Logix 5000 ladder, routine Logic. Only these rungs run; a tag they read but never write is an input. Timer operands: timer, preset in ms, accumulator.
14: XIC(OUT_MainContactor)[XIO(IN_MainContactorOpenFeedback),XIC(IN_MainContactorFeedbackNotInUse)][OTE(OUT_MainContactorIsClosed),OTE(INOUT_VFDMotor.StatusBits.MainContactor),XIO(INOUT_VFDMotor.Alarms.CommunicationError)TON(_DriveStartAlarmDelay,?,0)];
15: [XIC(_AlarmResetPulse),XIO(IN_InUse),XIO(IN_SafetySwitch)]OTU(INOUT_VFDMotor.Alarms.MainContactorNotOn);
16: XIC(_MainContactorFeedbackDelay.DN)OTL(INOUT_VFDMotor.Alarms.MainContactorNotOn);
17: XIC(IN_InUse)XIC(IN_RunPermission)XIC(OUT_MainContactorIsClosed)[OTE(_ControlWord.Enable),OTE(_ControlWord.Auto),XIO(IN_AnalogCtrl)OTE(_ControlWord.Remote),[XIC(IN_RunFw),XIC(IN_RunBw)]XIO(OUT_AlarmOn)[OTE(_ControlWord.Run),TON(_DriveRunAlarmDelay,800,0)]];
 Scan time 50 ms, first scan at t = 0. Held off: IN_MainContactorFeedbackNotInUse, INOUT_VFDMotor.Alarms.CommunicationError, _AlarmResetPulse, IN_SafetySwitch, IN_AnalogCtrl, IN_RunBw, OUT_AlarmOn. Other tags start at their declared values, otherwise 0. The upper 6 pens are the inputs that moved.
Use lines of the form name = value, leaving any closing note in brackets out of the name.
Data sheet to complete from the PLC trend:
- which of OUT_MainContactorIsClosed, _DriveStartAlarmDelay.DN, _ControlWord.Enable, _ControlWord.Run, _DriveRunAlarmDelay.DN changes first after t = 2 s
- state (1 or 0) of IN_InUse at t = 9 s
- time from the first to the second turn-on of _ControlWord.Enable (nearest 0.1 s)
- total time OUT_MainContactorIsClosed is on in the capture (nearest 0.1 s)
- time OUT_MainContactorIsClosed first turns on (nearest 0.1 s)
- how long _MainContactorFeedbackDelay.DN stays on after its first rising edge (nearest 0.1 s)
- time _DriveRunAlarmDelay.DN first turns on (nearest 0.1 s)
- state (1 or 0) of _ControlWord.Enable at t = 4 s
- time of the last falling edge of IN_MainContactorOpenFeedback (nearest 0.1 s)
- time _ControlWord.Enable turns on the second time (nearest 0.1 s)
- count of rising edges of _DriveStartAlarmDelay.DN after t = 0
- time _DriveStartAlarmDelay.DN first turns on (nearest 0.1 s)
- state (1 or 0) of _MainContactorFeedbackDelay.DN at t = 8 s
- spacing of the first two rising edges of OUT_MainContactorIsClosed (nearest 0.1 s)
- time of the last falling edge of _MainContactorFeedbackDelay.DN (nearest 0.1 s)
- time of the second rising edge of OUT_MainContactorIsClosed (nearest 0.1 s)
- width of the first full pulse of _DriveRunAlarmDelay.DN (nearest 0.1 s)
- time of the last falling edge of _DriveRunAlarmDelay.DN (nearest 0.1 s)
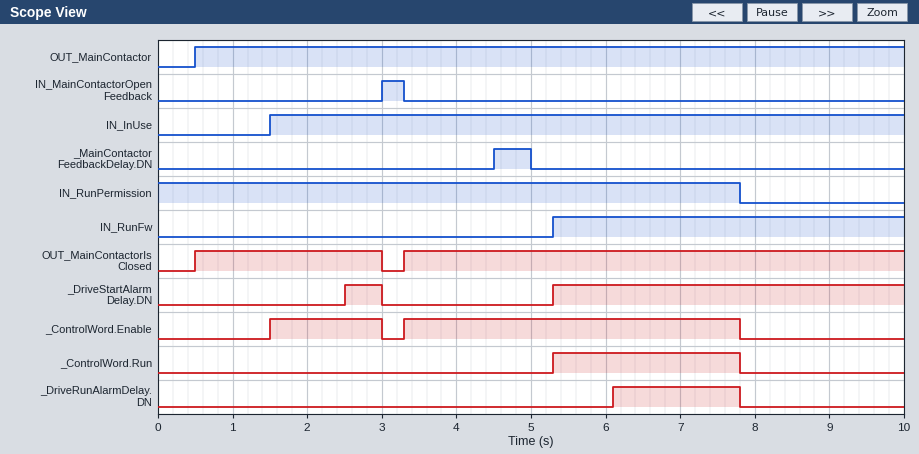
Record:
which of OUT_MainContactorIsClosed, _DriveStartAlarmDelay.DN, _ControlWord.Enable, _ControlWord.Run, _DriveRunAlarmDelay.DN changes first after t = 2 s = _DriveStartAlarmDelay.DN
state (1 or 0) of IN_InUse at t = 9 s = 1
time from the first to the second turn-on of _ControlWord.Enable = 1.8 s
total time OUT_MainContactorIsClosed is on in the capture = 9.2 s
time OUT_MainContactorIsClosed first turns on = 0.5 s
how long _MainContactorFeedbackDelay.DN stays on after its first rising edge = 0.5 s
time _DriveRunAlarmDelay.DN first turns on = 6.1 s
state (1 or 0) of _ControlWord.Enable at t = 4 s = 1
time of the last falling edge of IN_MainContactorOpenFeedback = 3.3 s
time _ControlWord.Enable turns on the second time = 3.3 s
count of rising edges of _DriveStartAlarmDelay.DN after t = 0 = 2
time _DriveStartAlarmDelay.DN first turns on = 2.5 s
state (1 or 0) of _MainContactorFeedbackDelay.DN at t = 8 s = 0
spacing of the first two rising edges of OUT_MainContactorIsClosed = 2.8 s
time of the last falling edge of _MainContactorFeedbackDelay.DN = 5.0 s
time of the second rising edge of OUT_MainContactorIsClosed = 3.3 s
width of the first full pulse of _DriveRunAlarmDelay.DN = 1.7 s
time of the last falling edge of _DriveRunAlarmDelay.DN = 7.8 s
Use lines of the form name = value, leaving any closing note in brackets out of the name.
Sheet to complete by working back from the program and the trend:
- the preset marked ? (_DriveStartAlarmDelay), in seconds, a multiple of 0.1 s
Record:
the preset marked ? (_DriveStartAlarmDelay), in seconds, a multiple of 0.1 s = 2.0 s
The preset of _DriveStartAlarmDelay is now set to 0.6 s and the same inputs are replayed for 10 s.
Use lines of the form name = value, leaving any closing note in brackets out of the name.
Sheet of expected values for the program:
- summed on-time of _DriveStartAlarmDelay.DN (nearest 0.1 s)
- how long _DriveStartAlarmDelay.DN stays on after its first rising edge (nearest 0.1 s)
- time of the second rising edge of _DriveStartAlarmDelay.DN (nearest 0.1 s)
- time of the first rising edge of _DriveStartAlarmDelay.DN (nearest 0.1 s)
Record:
summed on-time of _DriveStartAlarmDelay.DN = 8.0 s
how long _DriveStartAlarmDelay.DN stays on after its first rising edge = 1.9 s
time of the second rising edge of _DriveStartAlarmDelay.DN = 3.9 s
time of the first rising edge of _DriveStartAlarmDelay.DN = 1.1 s
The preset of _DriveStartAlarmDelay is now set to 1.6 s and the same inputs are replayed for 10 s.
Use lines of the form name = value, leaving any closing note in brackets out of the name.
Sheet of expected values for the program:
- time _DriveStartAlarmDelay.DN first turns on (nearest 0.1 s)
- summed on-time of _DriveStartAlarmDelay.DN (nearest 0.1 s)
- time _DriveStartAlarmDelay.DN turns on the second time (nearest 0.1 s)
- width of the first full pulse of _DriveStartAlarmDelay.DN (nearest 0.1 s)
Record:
time _DriveStartAlarmDelay.DN first turns on = 2.1 s
summed on-time of _DriveStartAlarmDelay.DN = 6.0 s
time _DriveStartAlarmDelay.DN turns on the second time = 4.9 s
width of the first full pulse of _DriveStartAlarmDelay.DN = 0.9 s
